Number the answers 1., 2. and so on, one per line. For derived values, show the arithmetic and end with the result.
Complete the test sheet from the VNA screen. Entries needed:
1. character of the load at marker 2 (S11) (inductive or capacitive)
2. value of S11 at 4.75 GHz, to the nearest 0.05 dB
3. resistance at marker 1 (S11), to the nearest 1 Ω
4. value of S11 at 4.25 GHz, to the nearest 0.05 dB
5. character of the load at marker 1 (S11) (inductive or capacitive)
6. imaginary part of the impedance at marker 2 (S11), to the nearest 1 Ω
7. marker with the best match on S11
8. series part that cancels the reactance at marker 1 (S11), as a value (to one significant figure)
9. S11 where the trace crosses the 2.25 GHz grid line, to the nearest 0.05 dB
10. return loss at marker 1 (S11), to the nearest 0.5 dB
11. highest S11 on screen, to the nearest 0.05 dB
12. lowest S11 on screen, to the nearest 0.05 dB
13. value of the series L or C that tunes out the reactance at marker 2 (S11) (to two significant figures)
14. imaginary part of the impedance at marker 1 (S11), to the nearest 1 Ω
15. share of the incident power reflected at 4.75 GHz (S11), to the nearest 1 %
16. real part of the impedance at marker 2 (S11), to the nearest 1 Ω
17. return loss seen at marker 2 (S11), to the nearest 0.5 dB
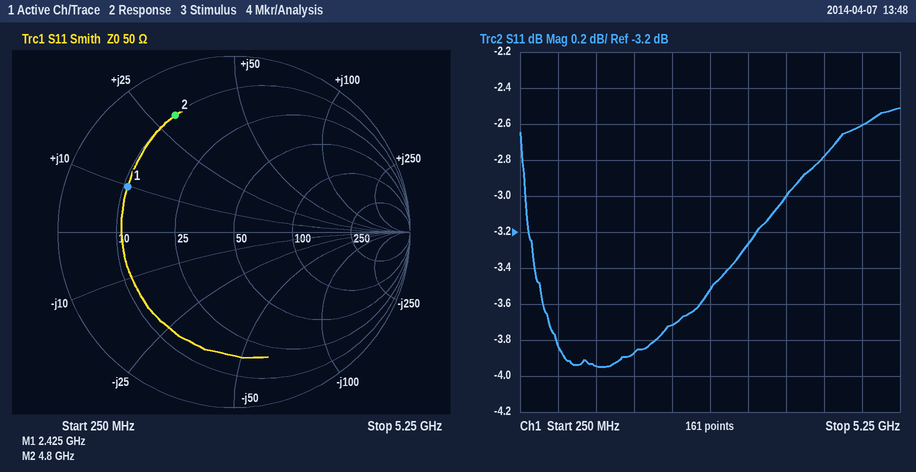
1. inductive
2. -2.60 dB
3. 11 Ω
4. -2.80 dB
5. inductive
6. +30 Ω
7. marker 1
8. C = 1/(2π × 2.425 GHz × 10 Ω) ≈ 7 pF
9. -3.70 dB
10. 3.5 dB
11. -2.50 dB
12. -3.95 dB
13. C = 1/(2π × 4.8 GHz × 30 Ω) ≈ 1.1 pF
14. +10 Ω
15. 10^(-2.6/10) ≈ 55 %
16. 10 Ω
17. 2.5 dB
